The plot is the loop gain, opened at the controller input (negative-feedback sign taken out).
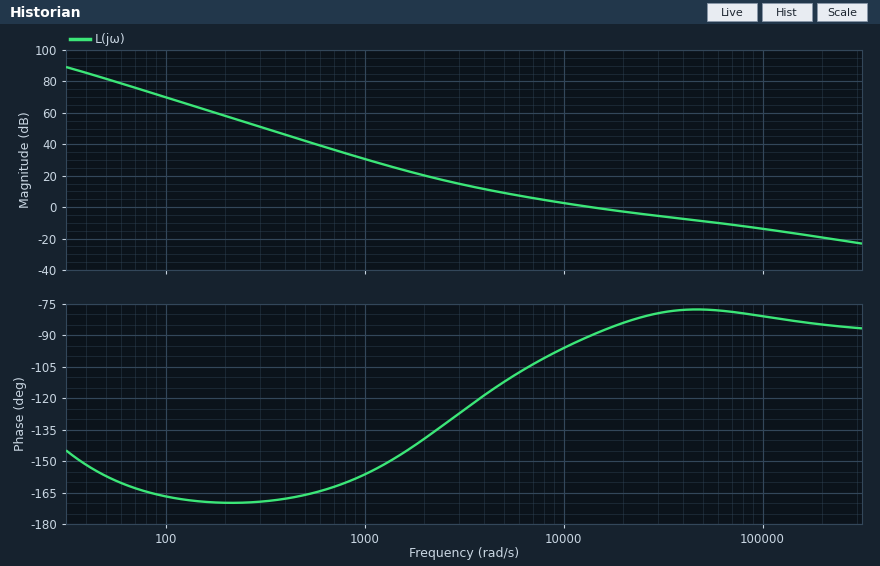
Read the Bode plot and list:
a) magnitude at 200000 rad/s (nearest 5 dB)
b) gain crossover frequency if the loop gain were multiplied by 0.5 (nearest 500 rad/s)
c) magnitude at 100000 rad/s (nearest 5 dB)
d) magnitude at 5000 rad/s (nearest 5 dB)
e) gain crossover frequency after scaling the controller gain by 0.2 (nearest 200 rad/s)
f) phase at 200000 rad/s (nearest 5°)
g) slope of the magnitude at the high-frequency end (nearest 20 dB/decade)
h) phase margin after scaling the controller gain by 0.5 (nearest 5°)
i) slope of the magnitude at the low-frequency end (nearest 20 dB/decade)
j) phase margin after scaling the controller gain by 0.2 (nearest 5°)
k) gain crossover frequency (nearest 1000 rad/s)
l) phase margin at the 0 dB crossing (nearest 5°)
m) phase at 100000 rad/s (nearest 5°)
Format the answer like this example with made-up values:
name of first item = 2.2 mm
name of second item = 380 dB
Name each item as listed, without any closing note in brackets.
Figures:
magnitude at 200000 rad/s = -20 dB
gain crossover frequency if the loop gain were multiplied by 0.5 = 7000 rad/s
magnitude at 100000 rad/s = -15 dB
magnitude at 5000 rad/s = 10 dB
gain crossover frequency after scaling the controller gain by 0.2 = 3200 rad/s
phase at 200000 rad/s = -85°
slope of the magnitude at the high-frequency end = -20 dB/decade
phase margin after scaling the controller gain by 0.5 = 75°
slope of the magnitude at the low-frequency end = -40 dB/decade
phase margin after scaling the controller gain by 0.2 = 55°
gain crossover frequency = 14000 rad/s
phase margin at the 0 dB crossing = 90°
phase at 100000 rad/s = -80°
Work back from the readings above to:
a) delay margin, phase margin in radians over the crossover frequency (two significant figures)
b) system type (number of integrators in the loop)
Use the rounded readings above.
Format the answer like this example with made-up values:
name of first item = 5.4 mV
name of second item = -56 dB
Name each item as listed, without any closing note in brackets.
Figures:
delay margin, phase margin in radians over the crossover frequency = 0.00011 s
system type = 2
